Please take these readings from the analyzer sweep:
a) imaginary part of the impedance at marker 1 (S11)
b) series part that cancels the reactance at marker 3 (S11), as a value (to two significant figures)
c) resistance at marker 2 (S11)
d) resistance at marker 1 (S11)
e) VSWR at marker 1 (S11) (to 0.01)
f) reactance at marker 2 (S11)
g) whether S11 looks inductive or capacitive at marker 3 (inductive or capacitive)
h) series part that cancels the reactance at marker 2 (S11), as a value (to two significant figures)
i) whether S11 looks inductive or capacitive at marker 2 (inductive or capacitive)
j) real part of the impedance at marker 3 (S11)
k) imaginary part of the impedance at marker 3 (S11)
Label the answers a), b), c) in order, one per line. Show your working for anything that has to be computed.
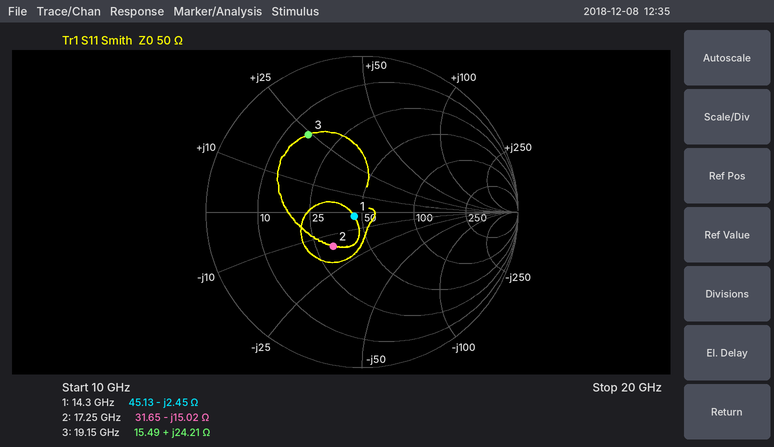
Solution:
a) -2.45 Ω
b) C = 1/(2π × 19.15 GHz × 24.21 Ω) ≈ 343 fF, so 340 fF to two significant figures
c) 31.65 Ω
d) 45.13 Ω
e) 1.12
f) -15.02 Ω
g) inductive
h) L = 15.02 Ω/(2π × 17.25 GHz) ≈ 139 pH, so 140 pH to two significant figures
i) capacitive
j) 15.49 Ω
k) +24.21 Ω
